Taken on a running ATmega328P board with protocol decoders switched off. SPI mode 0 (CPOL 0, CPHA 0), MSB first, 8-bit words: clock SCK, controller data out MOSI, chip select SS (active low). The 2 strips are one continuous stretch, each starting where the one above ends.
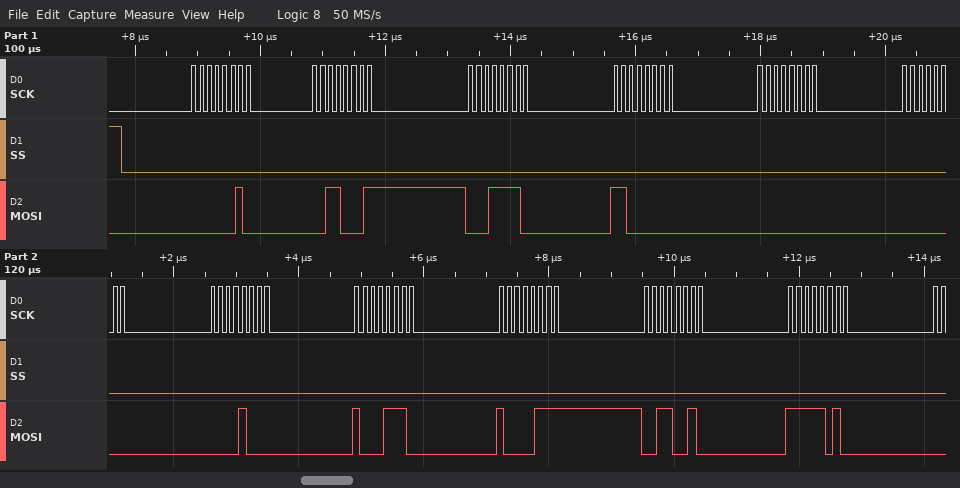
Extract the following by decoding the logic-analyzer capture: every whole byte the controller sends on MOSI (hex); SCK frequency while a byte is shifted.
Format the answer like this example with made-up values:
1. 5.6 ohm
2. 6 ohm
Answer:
1. 0x02 0x31 0x1E 0xC0 0x00 0x00 0x08 0x8E 0x87 0x32 0xFA
2. 8 MHz
